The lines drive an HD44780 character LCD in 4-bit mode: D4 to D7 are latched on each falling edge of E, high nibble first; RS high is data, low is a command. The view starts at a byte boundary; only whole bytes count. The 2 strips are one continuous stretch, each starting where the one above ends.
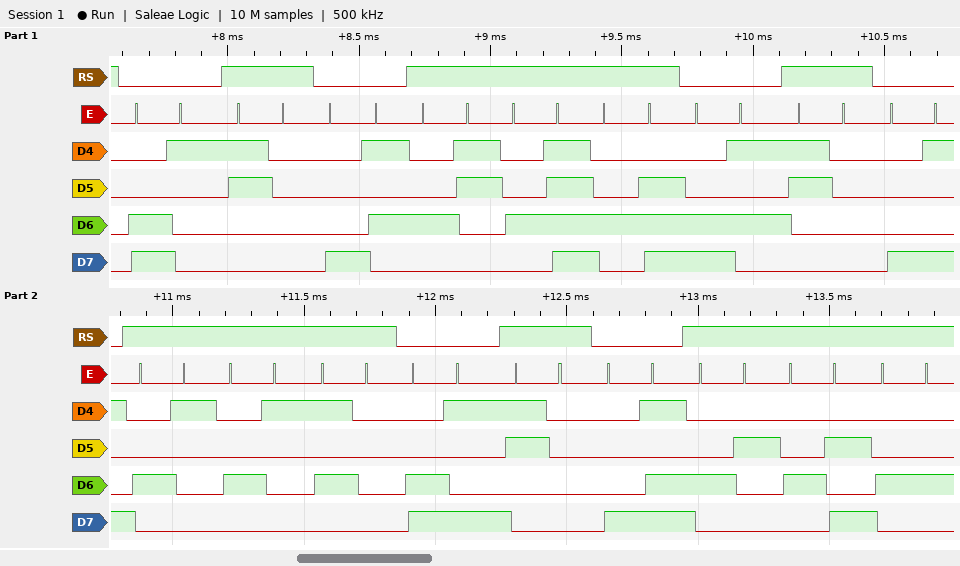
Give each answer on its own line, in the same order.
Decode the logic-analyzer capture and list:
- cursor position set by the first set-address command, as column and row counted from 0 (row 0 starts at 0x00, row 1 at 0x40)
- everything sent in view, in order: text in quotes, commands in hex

column 1, row 1
0xC1 "0" 0x85 "CON" 0xC5 "0" 0x89 "AAP" 0xC9 "0" 0x8D "BJD"
